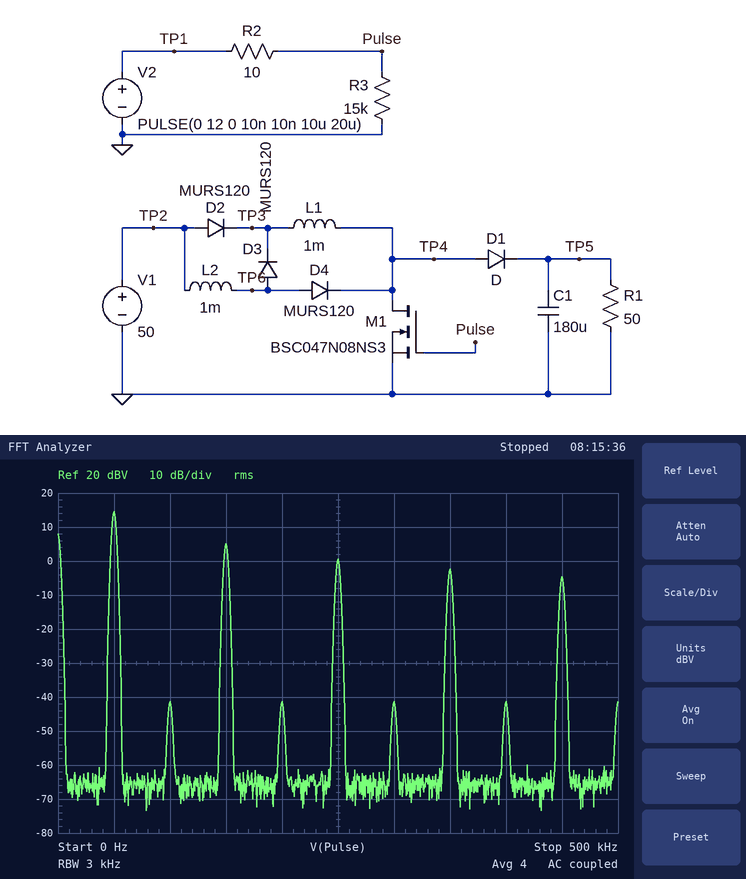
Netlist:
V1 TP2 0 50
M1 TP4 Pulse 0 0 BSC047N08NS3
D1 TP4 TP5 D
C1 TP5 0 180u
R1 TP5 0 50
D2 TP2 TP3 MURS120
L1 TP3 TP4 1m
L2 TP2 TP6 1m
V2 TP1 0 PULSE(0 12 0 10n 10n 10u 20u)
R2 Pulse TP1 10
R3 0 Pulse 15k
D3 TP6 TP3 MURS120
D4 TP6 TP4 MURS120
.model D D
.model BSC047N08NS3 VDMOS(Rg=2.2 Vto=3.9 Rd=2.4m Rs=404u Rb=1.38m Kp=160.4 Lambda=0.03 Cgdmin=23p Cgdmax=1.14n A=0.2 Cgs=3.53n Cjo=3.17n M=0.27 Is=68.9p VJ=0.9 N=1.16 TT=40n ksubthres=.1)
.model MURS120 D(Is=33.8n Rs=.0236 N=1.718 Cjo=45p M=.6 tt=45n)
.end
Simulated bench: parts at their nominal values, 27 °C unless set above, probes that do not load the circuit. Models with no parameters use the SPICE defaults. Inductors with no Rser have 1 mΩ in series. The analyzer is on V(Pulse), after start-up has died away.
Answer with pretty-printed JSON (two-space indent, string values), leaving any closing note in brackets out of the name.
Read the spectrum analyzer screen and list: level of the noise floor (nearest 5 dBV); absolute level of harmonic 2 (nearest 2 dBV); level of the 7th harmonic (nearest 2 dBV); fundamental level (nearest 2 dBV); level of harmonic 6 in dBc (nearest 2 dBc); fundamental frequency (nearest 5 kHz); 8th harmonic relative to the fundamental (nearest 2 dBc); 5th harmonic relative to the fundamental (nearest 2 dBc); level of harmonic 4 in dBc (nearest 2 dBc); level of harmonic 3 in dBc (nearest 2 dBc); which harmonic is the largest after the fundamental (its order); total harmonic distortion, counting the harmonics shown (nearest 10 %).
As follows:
{
  "level of the noise floor": "-65 dBV",
  "absolute level of harmonic 2": "-42 dBV",
  "level of the 7th harmonic": "-2 dBV",
  "fundamental level": "14 dBV",
  "level of harmonic 6 in dBc": "-56 dBc",
  "fundamental frequency": "50 kHz",
  "8th harmonic relative to the fundamental": "-56 dBc",
  "5th harmonic relative to the fundamental": "-14 dBc",
  "level of harmonic 4 in dBc": "-56 dBc",
  "level of harmonic 3 in dBc": "-10 dBc",
  "which harmonic is the largest after the fundamental": "3",
  "total harmonic distortion, counting the harmonics shown": "40 %"
}
